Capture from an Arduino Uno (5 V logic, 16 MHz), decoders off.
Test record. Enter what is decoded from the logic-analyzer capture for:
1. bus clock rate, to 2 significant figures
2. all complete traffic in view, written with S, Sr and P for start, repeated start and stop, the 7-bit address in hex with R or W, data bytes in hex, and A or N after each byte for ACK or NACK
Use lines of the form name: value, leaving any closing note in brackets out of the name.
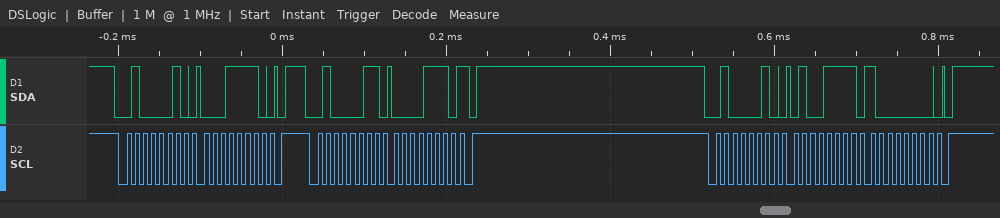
bus clock rate, to 2 significant figures: 100 kHz
all complete traffic in view, written with S, Sr and P for start, repeated start and stop, the 7-bit address in hex with R or W, data bytes in hex, and A or N after each byte for ACK or NACK: S 21W A 1E A P S 21R A 0E N P S 21W A 4F A 80 A P
